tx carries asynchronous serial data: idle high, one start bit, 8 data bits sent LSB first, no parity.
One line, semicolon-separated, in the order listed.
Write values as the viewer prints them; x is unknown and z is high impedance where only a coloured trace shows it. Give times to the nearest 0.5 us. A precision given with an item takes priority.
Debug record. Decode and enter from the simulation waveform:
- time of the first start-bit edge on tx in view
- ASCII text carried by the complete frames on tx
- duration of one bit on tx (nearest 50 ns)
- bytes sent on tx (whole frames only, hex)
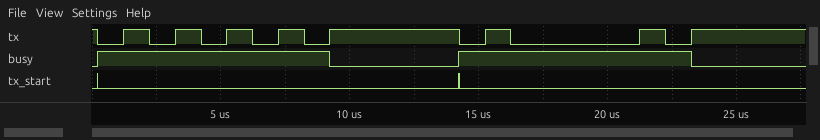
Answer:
0 us; "UA"; 1000 ns; 55, 41
